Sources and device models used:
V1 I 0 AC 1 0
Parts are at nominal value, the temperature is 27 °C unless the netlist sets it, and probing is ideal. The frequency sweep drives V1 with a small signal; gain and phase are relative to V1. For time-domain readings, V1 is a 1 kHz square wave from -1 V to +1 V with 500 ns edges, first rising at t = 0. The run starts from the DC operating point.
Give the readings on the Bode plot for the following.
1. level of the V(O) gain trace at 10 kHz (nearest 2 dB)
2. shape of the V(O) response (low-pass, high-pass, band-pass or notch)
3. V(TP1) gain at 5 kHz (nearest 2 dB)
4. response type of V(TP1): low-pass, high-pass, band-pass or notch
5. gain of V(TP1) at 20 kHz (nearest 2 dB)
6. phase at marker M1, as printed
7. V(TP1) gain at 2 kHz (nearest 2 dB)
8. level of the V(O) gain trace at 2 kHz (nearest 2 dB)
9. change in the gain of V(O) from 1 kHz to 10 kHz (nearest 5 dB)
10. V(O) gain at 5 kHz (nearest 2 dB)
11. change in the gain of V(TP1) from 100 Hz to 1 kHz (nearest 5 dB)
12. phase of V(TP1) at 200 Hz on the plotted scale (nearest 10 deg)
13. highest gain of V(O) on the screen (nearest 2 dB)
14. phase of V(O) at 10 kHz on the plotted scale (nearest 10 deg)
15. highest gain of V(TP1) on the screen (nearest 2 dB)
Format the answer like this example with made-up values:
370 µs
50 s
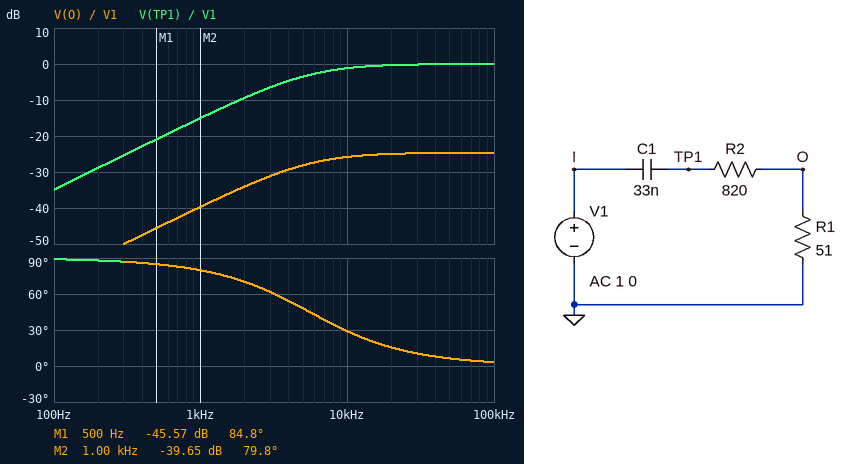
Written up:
-26 dB
high-pass
-4 dB
high-pass
0 dB
84.8 deg
-10 dB
-34 dB
15 dB
-28 dB
20 dB
90 deg
-24 dB
30 deg
0 dB
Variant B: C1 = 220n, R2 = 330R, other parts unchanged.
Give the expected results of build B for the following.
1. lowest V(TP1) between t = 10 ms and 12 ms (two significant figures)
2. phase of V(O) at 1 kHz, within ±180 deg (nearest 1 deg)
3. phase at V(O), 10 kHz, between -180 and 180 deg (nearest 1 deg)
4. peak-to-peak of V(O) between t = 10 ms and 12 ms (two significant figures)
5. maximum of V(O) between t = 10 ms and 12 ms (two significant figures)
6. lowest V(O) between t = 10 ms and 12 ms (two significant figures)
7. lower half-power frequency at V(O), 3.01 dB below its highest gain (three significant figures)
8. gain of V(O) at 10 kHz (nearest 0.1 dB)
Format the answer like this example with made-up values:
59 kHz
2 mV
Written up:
-2.0 V
62 deg
11 deg
530 mV
270 mV
-270 mV
1.90 kHz
-17.6 dB
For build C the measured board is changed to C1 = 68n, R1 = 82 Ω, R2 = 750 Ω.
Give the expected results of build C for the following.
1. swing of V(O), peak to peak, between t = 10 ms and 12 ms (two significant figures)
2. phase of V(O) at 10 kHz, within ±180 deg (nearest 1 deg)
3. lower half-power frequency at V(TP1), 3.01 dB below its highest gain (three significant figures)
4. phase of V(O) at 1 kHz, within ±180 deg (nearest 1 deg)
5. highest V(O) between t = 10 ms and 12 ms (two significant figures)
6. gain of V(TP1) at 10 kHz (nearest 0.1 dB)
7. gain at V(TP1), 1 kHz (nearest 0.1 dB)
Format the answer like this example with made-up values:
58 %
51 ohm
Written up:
390 mV
16 deg
2.81 kHz
70 deg
200 mV
-0.3 dB
-9.5 dB
